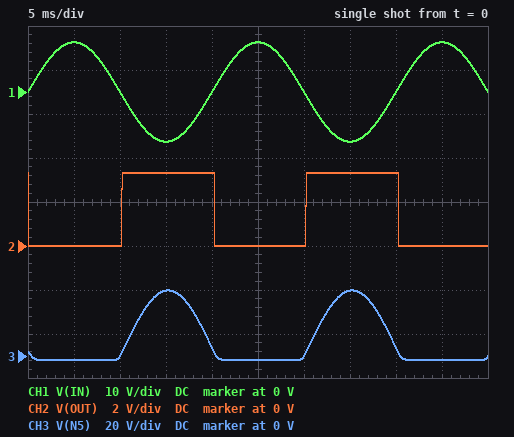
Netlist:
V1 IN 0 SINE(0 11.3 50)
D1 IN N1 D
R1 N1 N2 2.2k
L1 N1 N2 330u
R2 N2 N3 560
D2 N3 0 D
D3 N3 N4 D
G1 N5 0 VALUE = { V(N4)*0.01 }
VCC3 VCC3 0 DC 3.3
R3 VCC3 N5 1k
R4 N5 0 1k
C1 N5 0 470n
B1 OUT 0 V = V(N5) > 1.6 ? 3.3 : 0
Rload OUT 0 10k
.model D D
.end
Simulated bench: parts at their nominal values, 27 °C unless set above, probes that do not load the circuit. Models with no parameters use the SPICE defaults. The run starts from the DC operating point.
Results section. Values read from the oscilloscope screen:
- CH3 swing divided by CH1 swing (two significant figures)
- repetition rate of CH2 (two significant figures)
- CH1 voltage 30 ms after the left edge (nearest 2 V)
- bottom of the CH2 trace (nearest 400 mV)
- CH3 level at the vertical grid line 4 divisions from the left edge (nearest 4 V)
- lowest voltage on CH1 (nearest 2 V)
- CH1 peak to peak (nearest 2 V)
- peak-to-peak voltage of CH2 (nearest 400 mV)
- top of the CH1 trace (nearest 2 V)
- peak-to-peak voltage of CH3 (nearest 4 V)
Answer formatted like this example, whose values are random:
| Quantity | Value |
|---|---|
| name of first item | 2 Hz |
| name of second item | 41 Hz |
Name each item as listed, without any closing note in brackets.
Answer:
| Quantity | Value |
|---|---|
| CH3 swing divided by CH1 swing | 1.4 |
| repetition rate of CH2 | 50 Hz |
| CH1 voltage 30 ms after the left edge | 0 V |
| bottom of the CH2 trace | 0 V |
| CH3 level at the vertical grid line 4 divisions from the left edge | 4 V |
| lowest voltage on CH1 | -12 V |
| CH1 peak to peak | 22 V |
| peak-to-peak voltage of CH2 | 3.2 V |
| top of the CH1 trace | 12 V |
| peak-to-peak voltage of CH3 | 32 V |
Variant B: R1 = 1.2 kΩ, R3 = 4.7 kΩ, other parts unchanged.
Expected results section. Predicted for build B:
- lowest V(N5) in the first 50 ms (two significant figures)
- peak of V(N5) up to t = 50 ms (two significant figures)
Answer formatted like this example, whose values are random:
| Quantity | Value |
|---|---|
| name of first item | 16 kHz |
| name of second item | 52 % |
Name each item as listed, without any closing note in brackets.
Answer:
| Quantity | Value |
|---|---|
| lowest V(N5) in the first 50 ms | -5.4 V |
| peak of V(N5) up to t = 50 ms | 47 V |
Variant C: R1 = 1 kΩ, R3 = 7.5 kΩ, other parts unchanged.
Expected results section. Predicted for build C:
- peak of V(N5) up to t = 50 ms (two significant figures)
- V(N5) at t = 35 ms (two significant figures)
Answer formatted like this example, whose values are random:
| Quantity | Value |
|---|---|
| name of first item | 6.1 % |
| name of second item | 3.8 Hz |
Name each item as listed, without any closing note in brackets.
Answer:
| Quantity | Value |
|---|---|
| peak of V(N5) up to t = 50 ms | 50 V |
| V(N5) at t = 35 ms | 49 V |
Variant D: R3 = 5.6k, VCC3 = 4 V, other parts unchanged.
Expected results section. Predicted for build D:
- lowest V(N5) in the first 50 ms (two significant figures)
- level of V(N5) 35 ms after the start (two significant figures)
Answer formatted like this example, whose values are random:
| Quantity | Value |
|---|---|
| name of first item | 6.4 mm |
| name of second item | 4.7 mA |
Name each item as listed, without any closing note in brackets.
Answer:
| Quantity | Value |
|---|---|
| lowest V(N5) in the first 50 ms | -5.6 V |
| level of V(N5) 35 ms after the start | 48 V |
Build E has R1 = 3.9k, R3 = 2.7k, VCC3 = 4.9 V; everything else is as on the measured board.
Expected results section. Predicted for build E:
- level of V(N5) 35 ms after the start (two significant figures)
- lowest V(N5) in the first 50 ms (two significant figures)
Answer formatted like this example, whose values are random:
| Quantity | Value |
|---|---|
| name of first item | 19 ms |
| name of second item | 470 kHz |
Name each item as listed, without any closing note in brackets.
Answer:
| Quantity | Value |
|---|---|
| level of V(N5) 35 ms after the start | 42 V |
| lowest V(N5) in the first 50 ms | -4.0 V |
